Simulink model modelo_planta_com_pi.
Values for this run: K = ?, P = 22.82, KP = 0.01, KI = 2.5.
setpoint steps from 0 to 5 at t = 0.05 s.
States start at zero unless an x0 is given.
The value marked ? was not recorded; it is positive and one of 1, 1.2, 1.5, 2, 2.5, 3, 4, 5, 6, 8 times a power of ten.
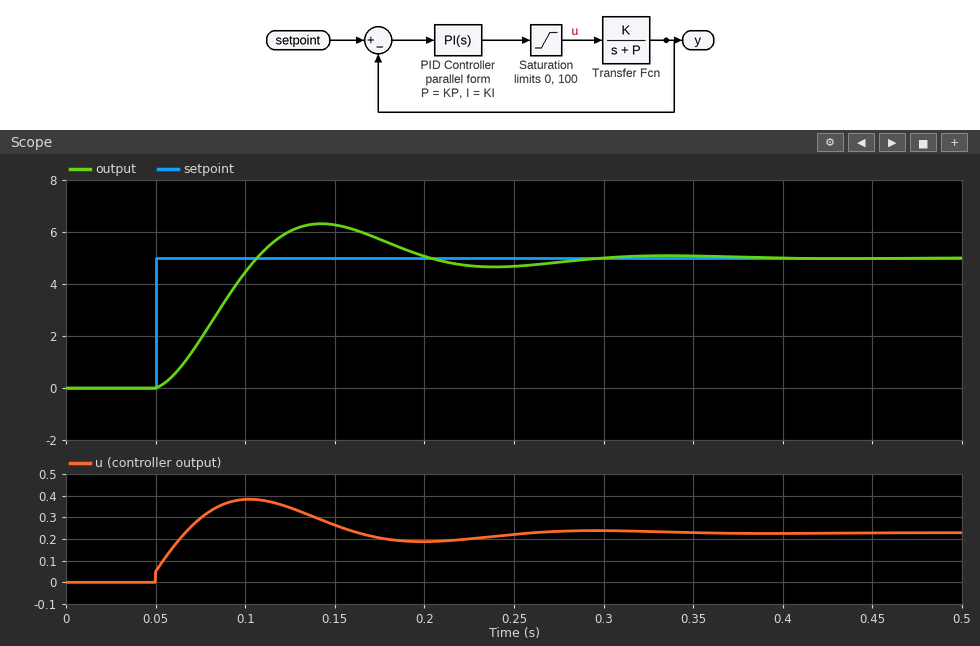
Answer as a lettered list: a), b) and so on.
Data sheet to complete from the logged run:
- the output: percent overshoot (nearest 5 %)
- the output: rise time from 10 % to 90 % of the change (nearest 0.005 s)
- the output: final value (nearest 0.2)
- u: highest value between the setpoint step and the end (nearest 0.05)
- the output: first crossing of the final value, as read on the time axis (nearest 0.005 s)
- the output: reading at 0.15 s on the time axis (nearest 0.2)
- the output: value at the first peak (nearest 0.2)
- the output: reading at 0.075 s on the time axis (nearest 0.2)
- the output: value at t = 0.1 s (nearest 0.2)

a) 25 %
b) 0.040 s
c) 5.0
d) 0.40
e) 0.105 s
f) 6.2
g) 6.4
h) 1.8
i) 4.4
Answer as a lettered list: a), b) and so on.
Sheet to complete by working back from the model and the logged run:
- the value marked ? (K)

a) 500
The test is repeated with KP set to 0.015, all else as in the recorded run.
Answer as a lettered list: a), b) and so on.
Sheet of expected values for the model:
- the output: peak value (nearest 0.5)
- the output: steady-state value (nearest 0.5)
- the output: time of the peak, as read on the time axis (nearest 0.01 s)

a) 6.0
b) 5.0
c) 0.14 s
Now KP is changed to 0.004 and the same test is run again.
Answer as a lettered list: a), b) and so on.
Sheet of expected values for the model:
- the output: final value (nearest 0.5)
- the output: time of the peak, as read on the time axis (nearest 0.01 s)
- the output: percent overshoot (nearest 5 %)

a) 5.0
b) 0.14 s
c) 30 %
